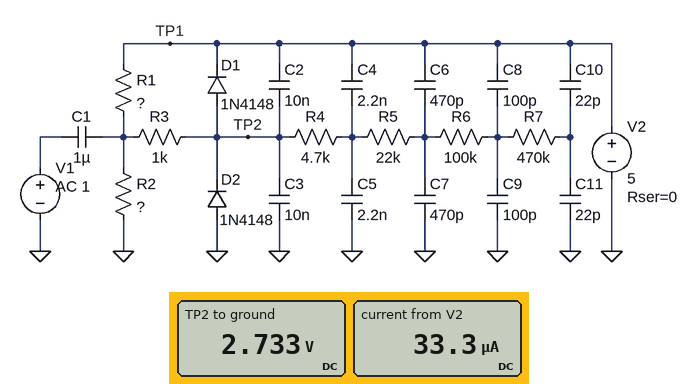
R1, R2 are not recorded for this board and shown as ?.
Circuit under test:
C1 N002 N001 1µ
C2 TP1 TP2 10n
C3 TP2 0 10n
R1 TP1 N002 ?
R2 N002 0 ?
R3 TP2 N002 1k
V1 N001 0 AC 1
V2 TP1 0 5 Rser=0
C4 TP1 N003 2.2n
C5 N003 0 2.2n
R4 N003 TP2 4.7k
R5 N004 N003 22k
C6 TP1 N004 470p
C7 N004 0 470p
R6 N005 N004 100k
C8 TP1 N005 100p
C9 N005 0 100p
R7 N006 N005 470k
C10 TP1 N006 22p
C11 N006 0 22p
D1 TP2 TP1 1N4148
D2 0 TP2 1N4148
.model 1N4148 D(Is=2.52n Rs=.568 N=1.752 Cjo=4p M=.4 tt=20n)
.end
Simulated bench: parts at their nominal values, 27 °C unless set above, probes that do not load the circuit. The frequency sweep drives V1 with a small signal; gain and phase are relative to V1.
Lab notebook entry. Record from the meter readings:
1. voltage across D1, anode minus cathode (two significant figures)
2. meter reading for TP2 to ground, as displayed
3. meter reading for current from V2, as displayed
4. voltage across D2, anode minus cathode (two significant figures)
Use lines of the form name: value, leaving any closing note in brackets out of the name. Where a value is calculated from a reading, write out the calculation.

voltage across D1, anode minus cathode: 2.733 V - 5 V = -2.3 V
meter reading for TP2 to ground, as displayed: 2.733 V
meter reading for current from V2, as displayed: 33.3 µA
voltage across D2, anode minus cathode: 0 V - 2.733 V = -2.7 V
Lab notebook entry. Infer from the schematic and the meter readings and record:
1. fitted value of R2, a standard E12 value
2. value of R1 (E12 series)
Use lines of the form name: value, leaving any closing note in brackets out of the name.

fitted value of R2, a standard E12 value: 82 kΩ
value of R1: 68 kΩ
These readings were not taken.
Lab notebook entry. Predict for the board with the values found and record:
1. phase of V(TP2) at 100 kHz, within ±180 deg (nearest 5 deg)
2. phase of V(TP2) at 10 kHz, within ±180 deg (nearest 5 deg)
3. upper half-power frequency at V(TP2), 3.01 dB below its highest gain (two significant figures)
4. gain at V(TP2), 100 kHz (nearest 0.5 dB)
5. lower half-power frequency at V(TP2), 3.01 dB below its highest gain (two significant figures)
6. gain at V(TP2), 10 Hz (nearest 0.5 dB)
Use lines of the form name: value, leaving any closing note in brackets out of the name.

phase of V(TP2) at 100 kHz, within ±180 deg: -85 deg
phase of V(TP2) at 10 kHz, within ±180 deg: -50 deg
upper half-power frequency at V(TP2), 3.01 dB below its highest gain: 6.6 kHz
gain at V(TP2), 100 kHz: -22.0 dB
lower half-power frequency at V(TP2), 3.01 dB below its highest gain: 4.2 Hz
gain at V(TP2), 10 Hz: -1.0 dB
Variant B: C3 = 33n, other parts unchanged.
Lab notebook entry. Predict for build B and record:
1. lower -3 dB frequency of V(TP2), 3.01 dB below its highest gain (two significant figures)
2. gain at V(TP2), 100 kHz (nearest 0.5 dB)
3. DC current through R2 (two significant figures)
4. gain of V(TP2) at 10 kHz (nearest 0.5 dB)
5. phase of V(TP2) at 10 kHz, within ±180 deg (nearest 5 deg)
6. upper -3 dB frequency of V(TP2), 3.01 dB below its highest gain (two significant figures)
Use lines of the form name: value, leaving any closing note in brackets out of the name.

lower -3 dB frequency of V(TP2), 3.01 dB below its highest gain: 4.1 Hz
gain at V(TP2), 100 kHz: -28.5 dB
DC current through R2: 33 µA
gain of V(TP2) at 10 kHz: -9.5 dB
phase of V(TP2) at 10 kHz, within ±180 deg: -65 deg
upper -3 dB frequency of V(TP2), 3.01 dB below its highest gain: 3.4 kHz
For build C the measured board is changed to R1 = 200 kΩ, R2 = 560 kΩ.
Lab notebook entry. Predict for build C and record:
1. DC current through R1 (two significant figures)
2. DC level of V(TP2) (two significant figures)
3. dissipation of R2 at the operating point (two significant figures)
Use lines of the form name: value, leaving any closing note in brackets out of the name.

DC current through R1: 6.6 µA
DC level of V(TP2): 3.7 V
dissipation of R2 at the operating point: 24 µW
